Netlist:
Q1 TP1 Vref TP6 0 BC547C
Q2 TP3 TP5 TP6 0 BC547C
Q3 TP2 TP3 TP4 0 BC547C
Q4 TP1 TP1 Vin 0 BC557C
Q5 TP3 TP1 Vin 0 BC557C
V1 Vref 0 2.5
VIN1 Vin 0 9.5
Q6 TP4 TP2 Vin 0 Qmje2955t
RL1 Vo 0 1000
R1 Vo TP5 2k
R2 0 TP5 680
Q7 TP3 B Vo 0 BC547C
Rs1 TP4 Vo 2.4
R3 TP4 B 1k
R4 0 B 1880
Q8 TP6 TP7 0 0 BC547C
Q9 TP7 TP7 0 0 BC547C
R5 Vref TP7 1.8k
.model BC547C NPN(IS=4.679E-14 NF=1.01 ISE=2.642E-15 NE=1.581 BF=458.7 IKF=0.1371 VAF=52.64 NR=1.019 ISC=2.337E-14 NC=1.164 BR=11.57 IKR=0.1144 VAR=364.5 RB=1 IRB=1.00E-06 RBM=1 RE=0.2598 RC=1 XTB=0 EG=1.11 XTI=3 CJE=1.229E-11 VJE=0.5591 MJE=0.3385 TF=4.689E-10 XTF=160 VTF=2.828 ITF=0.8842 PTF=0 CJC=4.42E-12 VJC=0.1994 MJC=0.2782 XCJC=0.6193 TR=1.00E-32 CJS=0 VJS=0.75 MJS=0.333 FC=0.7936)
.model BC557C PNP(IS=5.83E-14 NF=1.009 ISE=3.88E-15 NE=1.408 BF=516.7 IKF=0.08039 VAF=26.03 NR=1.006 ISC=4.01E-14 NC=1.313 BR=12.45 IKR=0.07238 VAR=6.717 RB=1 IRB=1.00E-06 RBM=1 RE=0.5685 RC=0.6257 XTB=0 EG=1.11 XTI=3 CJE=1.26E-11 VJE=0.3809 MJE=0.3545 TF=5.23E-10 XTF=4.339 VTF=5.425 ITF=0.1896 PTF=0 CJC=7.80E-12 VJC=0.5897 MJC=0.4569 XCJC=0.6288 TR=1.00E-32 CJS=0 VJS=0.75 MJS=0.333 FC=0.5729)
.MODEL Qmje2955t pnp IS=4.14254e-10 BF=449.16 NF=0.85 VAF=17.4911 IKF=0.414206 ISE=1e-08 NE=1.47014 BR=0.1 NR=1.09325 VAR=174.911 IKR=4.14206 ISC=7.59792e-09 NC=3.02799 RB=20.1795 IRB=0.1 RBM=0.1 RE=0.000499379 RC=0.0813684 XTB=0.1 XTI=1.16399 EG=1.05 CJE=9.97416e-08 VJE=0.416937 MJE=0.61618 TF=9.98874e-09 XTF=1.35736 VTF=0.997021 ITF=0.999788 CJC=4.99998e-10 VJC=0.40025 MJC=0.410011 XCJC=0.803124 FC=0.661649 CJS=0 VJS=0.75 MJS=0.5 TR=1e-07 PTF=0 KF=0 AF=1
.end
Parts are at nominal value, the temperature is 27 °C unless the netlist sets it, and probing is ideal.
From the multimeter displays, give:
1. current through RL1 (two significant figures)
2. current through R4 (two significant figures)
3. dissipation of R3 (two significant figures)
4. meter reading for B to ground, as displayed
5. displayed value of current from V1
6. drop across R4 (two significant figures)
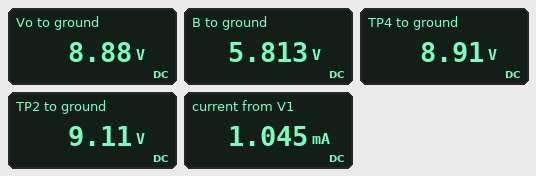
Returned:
8.9 mA
3.1 mA
9.6 mW
5.813 V
1.045 mA
5.8 V
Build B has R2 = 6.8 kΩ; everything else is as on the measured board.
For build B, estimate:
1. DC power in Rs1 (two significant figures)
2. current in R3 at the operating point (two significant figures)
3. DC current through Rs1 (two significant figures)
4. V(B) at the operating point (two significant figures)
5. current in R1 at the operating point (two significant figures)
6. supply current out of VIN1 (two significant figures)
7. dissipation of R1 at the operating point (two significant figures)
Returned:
31 µW
1.1 mA
3.6 mA
2.1 V
370 µA
5.8 mA
270 µW
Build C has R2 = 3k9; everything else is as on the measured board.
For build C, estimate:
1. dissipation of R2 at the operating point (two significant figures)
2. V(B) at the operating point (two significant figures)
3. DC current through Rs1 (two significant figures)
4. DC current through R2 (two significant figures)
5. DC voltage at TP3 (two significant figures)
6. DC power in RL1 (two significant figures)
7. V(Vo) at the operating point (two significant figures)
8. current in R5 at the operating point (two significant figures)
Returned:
1.6 mW
2.5 V
4.4 mA
640 µA
4.4 V
14 mW
3.8 V
1.0 mA
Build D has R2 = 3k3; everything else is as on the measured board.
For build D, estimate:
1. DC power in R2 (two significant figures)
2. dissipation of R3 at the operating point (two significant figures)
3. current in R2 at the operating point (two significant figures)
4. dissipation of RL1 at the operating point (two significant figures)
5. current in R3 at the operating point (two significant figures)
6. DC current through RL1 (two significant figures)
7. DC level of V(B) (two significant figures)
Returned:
1.9 mW
2.0 mW
760 µA
16 mW
1.4 mA
4.0 mA
2.6 V
